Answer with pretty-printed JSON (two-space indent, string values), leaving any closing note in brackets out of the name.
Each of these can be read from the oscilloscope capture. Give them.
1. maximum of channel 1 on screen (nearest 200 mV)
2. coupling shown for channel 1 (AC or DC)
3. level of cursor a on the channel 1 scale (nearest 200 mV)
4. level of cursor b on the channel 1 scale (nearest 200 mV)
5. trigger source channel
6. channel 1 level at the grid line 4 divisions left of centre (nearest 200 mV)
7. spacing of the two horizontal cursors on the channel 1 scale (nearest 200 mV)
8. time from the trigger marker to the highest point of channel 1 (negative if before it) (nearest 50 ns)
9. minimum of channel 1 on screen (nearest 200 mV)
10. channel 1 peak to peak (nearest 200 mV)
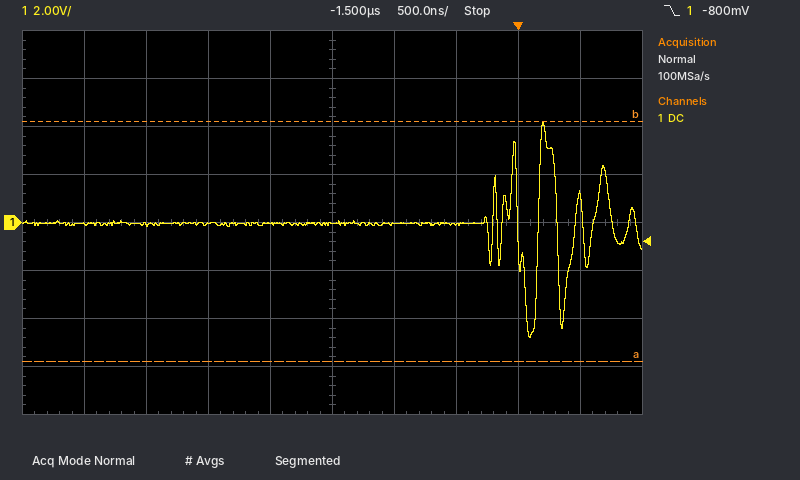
{
  "maximum of channel 1 on screen": "4.2 V",
  "coupling shown for channel 1": "DC",
  "level of cursor a on the channel 1 scale": "-5.8 V",
  "level of cursor b on the channel 1 scale": "4.2 V",
  "trigger source channel": "channel 1",
  "channel 1 level at the grid line 4 divisions left of centre": "0.0 V",
  "spacing of the two horizontal cursors on the channel 1 scale": "10.0 V",
  "time from the trigger marker to the highest point of channel 1 (negative if before it)": "+200 ns",
  "minimum of channel 1 on screen": "-4.8 V",
  "channel 1 peak to peak": "9.0 V"
}
